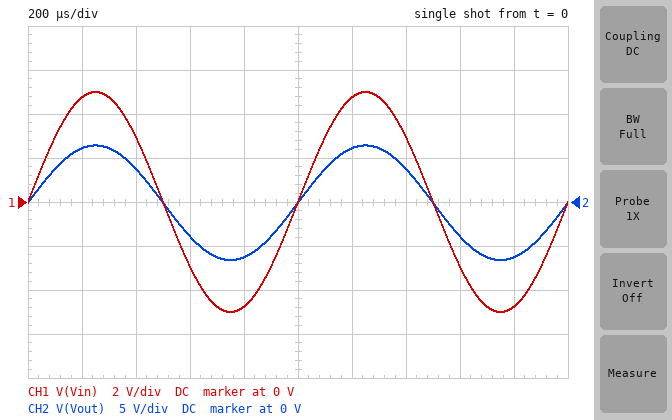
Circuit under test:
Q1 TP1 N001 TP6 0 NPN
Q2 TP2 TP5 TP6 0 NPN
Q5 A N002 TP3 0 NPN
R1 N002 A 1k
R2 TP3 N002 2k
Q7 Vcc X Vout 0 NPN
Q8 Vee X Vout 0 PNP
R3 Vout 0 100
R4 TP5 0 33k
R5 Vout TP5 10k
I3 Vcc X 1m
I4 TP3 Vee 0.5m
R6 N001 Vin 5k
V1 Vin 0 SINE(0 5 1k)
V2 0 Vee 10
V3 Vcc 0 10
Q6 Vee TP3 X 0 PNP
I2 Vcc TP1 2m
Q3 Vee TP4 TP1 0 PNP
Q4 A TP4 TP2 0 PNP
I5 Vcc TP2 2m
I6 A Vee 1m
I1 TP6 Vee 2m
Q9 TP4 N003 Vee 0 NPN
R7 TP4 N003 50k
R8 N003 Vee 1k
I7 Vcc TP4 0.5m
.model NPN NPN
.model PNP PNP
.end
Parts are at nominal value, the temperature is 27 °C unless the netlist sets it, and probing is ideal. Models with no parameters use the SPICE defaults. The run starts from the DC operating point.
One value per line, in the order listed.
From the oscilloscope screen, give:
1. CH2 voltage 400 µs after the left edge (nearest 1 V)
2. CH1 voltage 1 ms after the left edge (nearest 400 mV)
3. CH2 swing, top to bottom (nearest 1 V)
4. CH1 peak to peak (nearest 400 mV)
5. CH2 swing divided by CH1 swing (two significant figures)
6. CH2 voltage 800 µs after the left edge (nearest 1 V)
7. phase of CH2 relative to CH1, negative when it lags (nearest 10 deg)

4 V
0 V
13 V
10.0 V
1.3
-6 V
0 deg
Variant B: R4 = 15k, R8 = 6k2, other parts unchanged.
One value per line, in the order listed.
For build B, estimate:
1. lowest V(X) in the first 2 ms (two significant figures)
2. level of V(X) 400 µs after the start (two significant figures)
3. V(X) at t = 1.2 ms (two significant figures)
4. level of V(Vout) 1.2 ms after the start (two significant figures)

-9.3 V
-2.3 V
-2.2 V
-1.4 V
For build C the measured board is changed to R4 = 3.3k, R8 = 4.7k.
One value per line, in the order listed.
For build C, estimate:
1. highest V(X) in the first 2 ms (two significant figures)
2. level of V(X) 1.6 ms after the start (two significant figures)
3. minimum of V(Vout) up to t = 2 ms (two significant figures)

-170 mV
-10 V
-9.1 V
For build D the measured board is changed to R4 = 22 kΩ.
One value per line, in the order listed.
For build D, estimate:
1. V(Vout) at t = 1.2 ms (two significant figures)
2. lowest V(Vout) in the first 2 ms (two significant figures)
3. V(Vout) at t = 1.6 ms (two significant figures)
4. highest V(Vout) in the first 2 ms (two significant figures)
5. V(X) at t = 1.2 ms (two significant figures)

6.8 V
-7.4 V
-4.4 V
7.2 V
7.7 V
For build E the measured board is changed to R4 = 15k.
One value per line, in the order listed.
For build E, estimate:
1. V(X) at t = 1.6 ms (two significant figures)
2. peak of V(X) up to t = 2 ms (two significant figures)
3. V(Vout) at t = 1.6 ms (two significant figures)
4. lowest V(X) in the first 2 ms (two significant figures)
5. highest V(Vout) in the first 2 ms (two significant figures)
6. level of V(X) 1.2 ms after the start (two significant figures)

-5.9 V
9.1 V
-5.0 V
-9.3 V
8.2 V
8.7 V
